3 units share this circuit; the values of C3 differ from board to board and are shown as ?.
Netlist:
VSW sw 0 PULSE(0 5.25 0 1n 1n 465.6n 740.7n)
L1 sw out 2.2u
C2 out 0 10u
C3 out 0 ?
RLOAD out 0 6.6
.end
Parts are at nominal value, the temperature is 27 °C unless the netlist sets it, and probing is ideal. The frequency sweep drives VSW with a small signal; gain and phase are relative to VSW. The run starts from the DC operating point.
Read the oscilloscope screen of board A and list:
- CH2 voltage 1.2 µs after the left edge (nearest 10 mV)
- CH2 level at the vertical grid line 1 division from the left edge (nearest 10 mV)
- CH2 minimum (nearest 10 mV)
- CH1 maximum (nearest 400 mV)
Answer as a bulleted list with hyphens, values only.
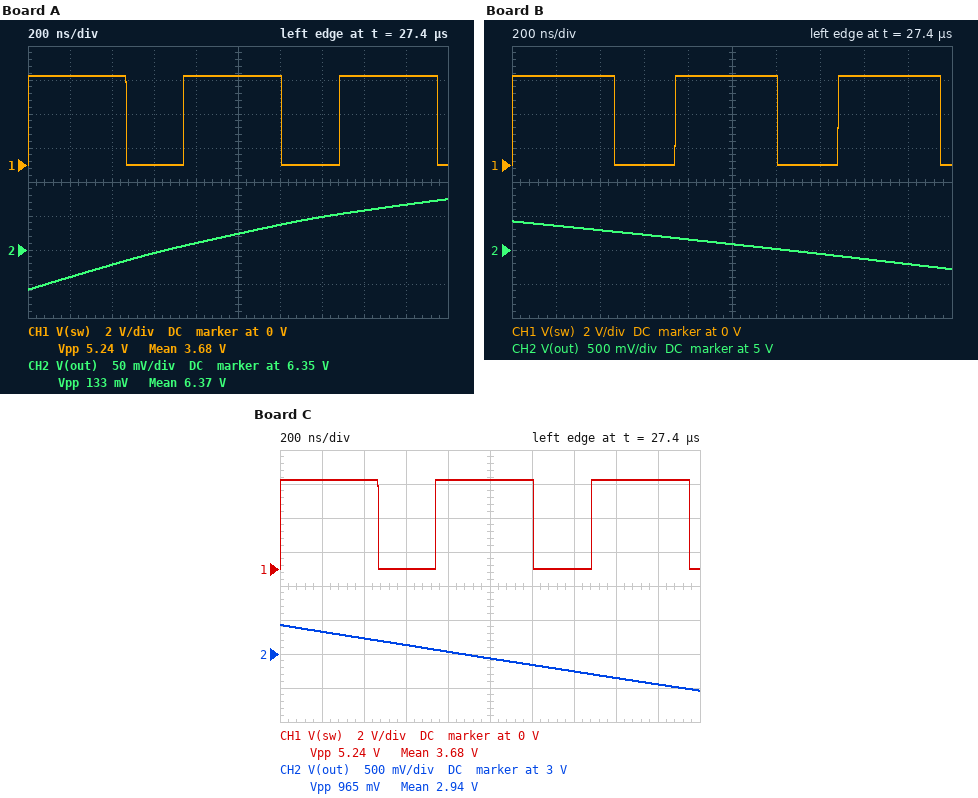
- 6.39 V
- 6.31 V
- 6.29 V
- 5.2 V
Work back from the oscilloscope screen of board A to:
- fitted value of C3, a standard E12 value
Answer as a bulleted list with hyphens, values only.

- 33 µF
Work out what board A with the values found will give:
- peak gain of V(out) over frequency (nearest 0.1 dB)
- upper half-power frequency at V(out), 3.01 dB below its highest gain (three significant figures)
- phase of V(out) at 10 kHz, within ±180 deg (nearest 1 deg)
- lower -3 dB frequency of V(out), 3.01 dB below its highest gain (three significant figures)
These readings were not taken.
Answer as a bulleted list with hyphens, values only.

- 29.3 dB
- 16.6 kHz
- -2 deg
- 16.1 kHz
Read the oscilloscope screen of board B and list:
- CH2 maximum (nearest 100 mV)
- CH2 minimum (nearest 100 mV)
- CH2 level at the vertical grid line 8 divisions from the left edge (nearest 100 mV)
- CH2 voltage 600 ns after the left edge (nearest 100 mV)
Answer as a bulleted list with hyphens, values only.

- 5.4 V
- 4.7 V
- 4.9 V
- 5.2 V
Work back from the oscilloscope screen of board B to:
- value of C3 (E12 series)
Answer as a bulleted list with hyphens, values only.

- 12 µF
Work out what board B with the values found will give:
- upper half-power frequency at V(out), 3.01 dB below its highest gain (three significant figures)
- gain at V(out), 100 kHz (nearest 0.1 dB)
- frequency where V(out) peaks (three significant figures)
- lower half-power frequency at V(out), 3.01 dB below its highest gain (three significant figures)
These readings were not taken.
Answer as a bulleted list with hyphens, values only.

- 23.4 kHz
- -25.2 dB
- 22.9 kHz
- 22.3 kHz
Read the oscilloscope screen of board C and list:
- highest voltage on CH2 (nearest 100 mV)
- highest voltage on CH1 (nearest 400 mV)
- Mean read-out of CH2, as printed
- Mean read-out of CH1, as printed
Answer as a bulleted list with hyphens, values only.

- 3.4 V
- 5.2 V
- 2.94 V
- 3.68 V
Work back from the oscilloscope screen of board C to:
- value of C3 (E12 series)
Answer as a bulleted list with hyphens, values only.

- 5.6 µF
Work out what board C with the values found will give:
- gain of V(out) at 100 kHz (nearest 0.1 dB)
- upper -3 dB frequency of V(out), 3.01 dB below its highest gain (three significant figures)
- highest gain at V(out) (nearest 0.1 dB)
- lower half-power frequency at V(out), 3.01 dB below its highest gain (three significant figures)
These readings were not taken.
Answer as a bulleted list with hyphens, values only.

- -22.0 dB
- 27.9 kHz
- 24.9 dB
- 26.4 kHz
